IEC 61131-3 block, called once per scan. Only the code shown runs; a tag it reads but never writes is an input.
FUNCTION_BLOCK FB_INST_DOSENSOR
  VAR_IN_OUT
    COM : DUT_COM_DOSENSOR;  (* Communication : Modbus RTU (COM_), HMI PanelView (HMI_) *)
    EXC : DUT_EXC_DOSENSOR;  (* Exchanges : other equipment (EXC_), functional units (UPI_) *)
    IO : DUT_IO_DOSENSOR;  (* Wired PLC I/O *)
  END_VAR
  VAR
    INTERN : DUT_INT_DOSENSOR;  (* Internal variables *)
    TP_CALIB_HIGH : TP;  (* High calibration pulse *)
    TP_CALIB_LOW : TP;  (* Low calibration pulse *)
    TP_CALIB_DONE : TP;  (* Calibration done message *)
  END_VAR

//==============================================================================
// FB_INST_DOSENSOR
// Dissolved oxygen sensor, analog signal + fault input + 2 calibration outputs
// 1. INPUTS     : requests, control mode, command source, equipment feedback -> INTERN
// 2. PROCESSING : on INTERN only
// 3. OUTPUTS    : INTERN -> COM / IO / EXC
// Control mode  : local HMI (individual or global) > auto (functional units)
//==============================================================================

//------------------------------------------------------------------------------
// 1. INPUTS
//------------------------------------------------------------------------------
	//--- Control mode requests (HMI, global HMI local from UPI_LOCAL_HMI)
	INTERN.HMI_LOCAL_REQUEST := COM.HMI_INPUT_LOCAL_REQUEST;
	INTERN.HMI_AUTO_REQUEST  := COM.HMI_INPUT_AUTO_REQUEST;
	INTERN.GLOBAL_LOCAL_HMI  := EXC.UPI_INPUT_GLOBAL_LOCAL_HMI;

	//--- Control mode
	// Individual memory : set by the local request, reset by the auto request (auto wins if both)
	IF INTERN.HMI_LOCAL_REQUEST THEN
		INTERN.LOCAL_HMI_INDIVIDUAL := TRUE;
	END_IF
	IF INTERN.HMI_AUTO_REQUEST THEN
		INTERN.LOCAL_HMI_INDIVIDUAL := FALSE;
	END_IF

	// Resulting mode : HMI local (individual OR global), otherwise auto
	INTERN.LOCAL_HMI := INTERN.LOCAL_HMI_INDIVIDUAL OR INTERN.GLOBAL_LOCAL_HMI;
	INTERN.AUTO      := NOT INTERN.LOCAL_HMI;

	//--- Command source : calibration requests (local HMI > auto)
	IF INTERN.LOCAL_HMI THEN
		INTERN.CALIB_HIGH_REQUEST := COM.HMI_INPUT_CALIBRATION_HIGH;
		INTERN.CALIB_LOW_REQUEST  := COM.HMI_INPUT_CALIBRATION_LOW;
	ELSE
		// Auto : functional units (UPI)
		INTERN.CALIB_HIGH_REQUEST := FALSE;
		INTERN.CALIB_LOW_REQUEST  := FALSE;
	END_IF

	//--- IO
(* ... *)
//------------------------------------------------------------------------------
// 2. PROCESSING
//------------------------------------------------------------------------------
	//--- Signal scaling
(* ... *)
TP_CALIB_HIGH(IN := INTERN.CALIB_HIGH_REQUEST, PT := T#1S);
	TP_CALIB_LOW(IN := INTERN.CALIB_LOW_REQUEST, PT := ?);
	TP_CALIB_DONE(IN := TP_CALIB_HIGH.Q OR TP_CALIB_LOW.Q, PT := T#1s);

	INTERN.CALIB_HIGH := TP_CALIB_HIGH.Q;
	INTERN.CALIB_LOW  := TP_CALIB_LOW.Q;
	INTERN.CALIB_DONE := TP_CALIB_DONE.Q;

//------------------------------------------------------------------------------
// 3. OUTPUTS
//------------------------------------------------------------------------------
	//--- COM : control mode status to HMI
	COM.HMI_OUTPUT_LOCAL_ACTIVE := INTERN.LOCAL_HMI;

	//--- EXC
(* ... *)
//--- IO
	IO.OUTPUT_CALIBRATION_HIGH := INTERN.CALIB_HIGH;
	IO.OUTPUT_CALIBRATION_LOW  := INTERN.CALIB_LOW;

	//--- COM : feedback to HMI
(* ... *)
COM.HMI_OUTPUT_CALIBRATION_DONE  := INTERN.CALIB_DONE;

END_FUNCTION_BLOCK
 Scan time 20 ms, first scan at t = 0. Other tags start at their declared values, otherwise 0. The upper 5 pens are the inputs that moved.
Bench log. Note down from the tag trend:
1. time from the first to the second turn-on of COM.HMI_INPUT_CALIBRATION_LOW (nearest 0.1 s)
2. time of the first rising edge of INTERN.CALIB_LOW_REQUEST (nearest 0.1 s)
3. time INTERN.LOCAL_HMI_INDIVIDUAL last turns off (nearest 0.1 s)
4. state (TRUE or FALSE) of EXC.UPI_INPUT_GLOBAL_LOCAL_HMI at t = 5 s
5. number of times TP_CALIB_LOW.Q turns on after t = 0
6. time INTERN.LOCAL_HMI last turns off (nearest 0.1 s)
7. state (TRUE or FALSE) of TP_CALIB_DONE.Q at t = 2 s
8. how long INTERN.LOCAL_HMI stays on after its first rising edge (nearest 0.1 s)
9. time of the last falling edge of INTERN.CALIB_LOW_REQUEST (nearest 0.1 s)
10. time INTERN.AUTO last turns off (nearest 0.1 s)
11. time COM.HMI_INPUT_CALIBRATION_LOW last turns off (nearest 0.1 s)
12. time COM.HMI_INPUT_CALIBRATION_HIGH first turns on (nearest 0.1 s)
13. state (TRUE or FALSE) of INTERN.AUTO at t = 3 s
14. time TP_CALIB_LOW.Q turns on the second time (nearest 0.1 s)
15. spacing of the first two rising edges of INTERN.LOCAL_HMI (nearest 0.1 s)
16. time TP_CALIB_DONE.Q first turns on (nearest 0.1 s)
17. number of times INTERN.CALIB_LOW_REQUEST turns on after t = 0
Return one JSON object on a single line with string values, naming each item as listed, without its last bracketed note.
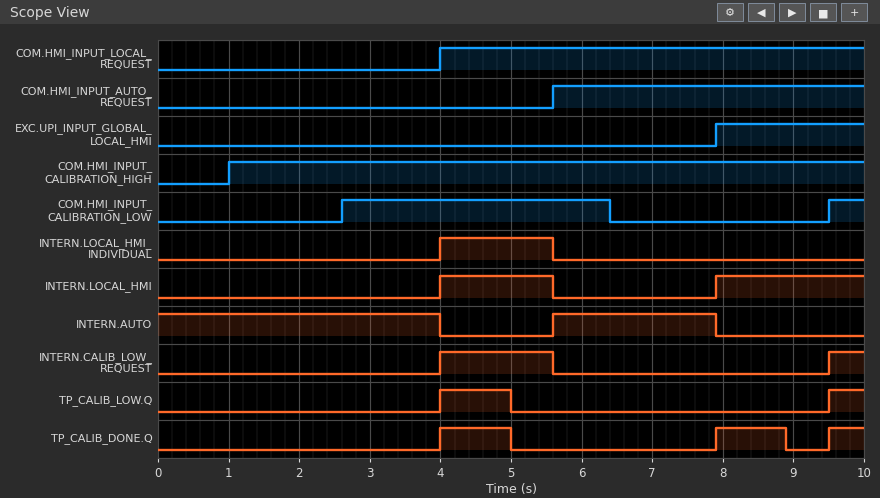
{"time from the first to the second turn-on of COM.HMI_INPUT_CALIBRATION_LOW": "6.9 s", "time of the first rising edge of INTERN.CALIB_LOW_REQUEST": "4.0 s", "time INTERN.LOCAL_HMI_INDIVIDUAL last turns off": "5.6 s", "state (TRUE or FALSE) of EXC.UPI_INPUT_GLOBAL_LOCAL_HMI at t = 5 s": "FALSE", "number of times TP_CALIB_LOW.Q turns on after t = 0": "2", "time INTERN.LOCAL_HMI last turns off": "5.6 s", "state (TRUE or FALSE) of TP_CALIB_DONE.Q at t = 2 s": "FALSE", "how long INTERN.LOCAL_HMI stays on after its first rising edge": "1.6 s", "time of the last falling edge of INTERN.CALIB_LOW_REQUEST": "5.6 s", "time INTERN.AUTO last turns off": "7.9 s", "time COM.HMI_INPUT_CALIBRATION_LOW last turns off": "6.4 s", "time COM.HMI_INPUT_CALIBRATION_HIGH first turns on": "1.0 s", "state (TRUE or FALSE) of INTERN.AUTO at t = 3 s": "TRUE", "time TP_CALIB_LOW.Q turns on the second time": "9.5 s", "spacing of the first two rising edges of INTERN.LOCAL_HMI": "3.9 s", "time TP_CALIB_DONE.Q first turns on": "4.0 s", "number of times INTERN.CALIB_LOW_REQUEST turns on after t = 0": "2"}
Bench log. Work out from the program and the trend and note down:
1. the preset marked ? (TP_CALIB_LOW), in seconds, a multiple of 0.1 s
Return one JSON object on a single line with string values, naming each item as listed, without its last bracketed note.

{"the preset marked ? (TP_CALIB_LOW), in seconds, a multiple of 0.1 s": "1.0 s"}
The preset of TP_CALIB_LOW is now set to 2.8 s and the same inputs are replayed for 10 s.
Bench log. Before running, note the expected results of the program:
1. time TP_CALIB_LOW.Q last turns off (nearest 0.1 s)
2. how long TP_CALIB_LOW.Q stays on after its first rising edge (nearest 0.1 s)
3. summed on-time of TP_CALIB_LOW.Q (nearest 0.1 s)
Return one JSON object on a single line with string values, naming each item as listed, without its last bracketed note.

{"time TP_CALIB_LOW.Q last turns off": "6.8 s", "how long TP_CALIB_LOW.Q stays on after its first rising edge": "2.8 s", "summed on-time of TP_CALIB_LOW.Q": "3.3 s"}
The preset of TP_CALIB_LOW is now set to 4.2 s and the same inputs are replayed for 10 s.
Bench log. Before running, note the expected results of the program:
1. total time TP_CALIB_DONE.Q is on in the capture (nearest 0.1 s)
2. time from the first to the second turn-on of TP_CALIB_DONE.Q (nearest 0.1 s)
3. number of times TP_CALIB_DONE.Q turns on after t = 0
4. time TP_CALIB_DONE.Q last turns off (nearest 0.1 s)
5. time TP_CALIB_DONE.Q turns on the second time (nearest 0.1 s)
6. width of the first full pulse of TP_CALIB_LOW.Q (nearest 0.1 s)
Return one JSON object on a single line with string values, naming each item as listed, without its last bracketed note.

{"total time TP_CALIB_DONE.Q is on in the capture": "1.5 s", "time from the first to the second turn-on of TP_CALIB_DONE.Q": "5.5 s", "number of times TP_CALIB_DONE.Q turns on after t = 0": "2", "time TP_CALIB_DONE.Q last turns off": "5.0 s", "time TP_CALIB_DONE.Q turns on the second time": "9.5 s", "width of the first full pulse of TP_CALIB_LOW.Q": "4.2 s"}
